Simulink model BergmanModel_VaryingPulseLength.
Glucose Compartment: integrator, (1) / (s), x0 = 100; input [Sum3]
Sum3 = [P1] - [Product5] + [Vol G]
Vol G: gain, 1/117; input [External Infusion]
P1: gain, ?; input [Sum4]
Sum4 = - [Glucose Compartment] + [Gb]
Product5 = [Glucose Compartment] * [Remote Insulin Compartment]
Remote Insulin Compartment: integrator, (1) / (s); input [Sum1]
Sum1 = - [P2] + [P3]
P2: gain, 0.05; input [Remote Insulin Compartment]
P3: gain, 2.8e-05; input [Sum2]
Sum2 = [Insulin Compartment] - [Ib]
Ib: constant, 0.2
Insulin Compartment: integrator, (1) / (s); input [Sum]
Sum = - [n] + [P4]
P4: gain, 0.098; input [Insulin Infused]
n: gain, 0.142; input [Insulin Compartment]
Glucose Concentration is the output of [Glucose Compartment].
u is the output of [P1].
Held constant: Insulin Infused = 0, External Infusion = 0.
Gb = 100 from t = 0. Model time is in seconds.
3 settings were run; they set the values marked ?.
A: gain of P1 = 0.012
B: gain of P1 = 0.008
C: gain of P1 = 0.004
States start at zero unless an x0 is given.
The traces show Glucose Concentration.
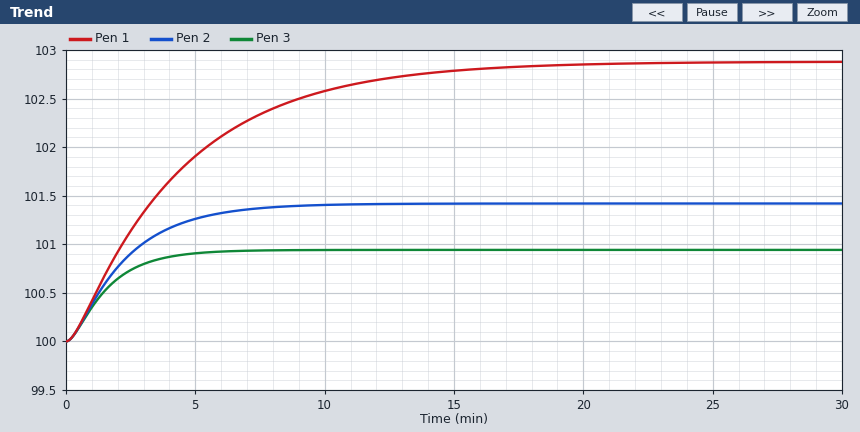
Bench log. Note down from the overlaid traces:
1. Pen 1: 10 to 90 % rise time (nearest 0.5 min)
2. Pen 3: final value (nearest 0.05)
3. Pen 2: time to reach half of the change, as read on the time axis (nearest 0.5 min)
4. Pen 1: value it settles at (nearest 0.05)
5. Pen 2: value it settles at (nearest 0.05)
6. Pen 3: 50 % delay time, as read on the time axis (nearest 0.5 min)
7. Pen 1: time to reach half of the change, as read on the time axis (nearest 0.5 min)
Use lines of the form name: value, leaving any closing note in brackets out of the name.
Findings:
Pen 1: 10 to 90 % rise time: 9.5 min
Pen 3: final value: 100.95
Pen 2: time to reach half of the change, as read on the time axis: 2.0 min
Pen 1: value it settles at: 102.90
Pen 2: value it settles at: 101.40
Pen 3: 50 % delay time, as read on the time axis: 1.5 min
Pen 1: time to reach half of the change, as read on the time axis: 3.5 min
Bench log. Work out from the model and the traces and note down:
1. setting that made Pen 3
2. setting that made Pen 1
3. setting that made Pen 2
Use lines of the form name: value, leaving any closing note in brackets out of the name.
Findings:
setting that made Pen 3: A
setting that made Pen 1: C
setting that made Pen 2: B
